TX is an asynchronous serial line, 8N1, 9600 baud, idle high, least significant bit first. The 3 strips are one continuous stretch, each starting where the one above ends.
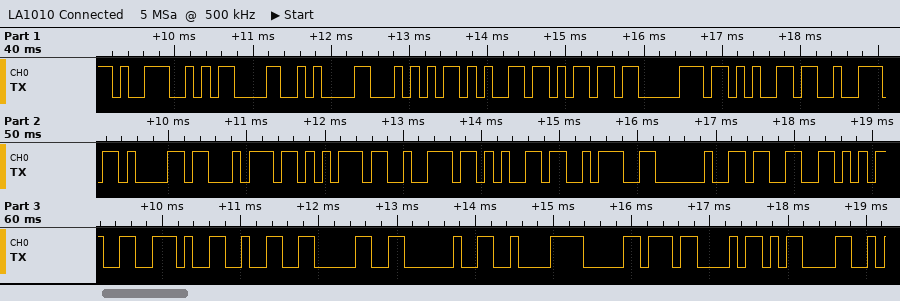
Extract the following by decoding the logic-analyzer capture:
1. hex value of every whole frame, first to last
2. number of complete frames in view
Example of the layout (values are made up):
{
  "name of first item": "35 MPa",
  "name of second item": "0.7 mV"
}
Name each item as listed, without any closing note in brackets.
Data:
{
  "hex value of every whole frame, first to last": "0x39 0x0D 0x0A 0x54 0x65 0x6D 0x70 0x65 0x72 0x61 0x74 0x75 0x72 0x65 0x3A 0x20 0x33 0x35 0x2E 0x32 0x30 0x20 0xC2 0xB0 0x43 0x0D",
  "number of complete frames in view": "26"
}
